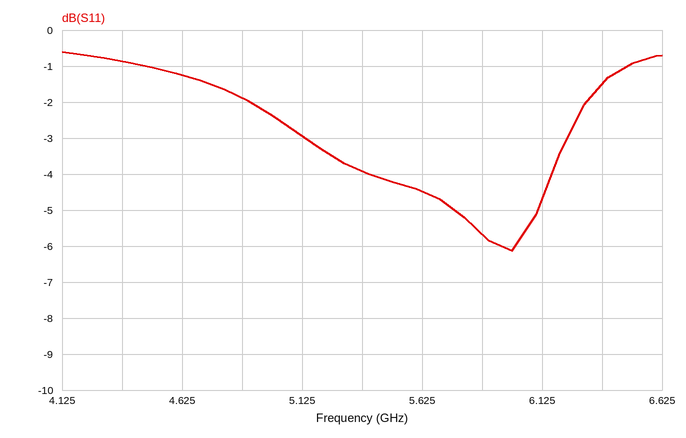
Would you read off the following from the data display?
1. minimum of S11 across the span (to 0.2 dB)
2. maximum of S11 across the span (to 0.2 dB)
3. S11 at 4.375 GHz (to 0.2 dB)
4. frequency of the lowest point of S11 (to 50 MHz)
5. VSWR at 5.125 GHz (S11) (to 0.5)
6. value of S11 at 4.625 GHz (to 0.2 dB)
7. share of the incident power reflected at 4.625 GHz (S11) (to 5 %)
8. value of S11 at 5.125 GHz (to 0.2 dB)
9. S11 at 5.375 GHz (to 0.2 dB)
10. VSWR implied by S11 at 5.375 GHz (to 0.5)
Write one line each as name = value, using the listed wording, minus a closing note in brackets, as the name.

minimum of S11 across the span = -6.2 dB
maximum of S11 across the span = -0.6 dB
S11 at 4.375 GHz = -0.8 dB
frequency of the lowest point of S11 = 6.00 GHz
VSWR at 5.125 GHz (S11) = 6.0
value of S11 at 4.625 GHz = -1.2 dB
share of the incident power reflected at 4.625 GHz (S11) = 75 %
value of S11 at 5.125 GHz = -3.0 dB
S11 at 5.375 GHz = -4.0 dB
VSWR implied by S11 at 5.375 GHz = 4.5
